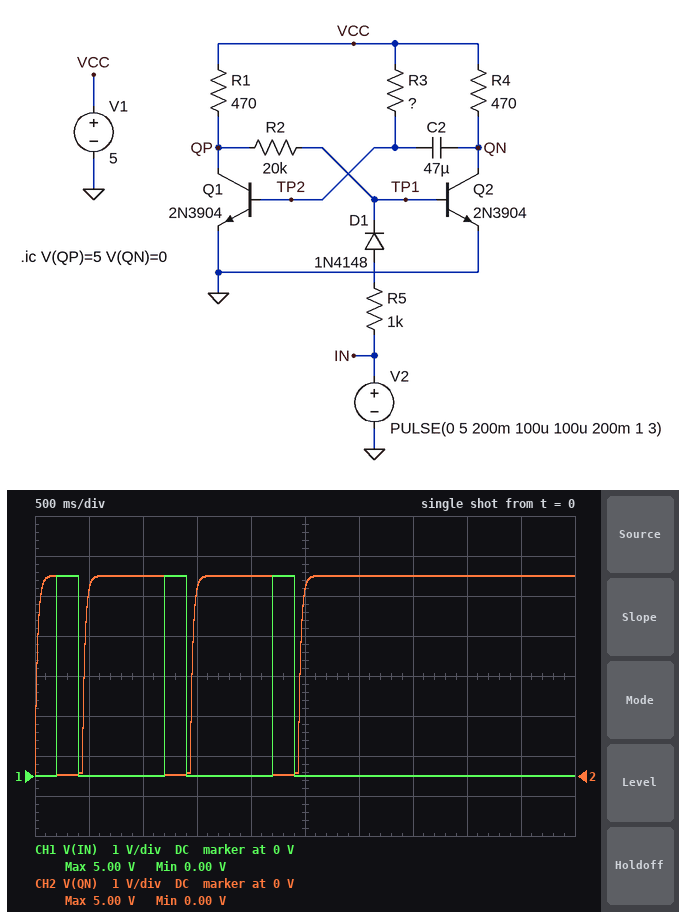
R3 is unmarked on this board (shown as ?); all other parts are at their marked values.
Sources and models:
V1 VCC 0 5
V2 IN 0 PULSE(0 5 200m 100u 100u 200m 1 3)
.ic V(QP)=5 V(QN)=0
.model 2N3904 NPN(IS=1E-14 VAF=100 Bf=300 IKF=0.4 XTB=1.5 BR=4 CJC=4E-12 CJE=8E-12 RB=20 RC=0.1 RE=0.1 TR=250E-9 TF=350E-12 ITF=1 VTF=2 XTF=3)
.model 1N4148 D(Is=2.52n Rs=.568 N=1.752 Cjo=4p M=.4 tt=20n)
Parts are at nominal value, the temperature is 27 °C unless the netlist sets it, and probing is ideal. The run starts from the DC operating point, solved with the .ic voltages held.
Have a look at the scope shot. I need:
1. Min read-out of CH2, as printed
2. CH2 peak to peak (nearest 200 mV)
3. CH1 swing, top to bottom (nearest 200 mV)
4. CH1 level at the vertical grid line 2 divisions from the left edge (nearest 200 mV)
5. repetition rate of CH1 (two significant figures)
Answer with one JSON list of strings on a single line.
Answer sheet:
["0.00 V", "5.0 V", "5.0 V", "0 V", "1.0 Hz"]
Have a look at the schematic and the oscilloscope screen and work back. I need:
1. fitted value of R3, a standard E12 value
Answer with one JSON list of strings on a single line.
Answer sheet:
["6.8 kΩ"]
